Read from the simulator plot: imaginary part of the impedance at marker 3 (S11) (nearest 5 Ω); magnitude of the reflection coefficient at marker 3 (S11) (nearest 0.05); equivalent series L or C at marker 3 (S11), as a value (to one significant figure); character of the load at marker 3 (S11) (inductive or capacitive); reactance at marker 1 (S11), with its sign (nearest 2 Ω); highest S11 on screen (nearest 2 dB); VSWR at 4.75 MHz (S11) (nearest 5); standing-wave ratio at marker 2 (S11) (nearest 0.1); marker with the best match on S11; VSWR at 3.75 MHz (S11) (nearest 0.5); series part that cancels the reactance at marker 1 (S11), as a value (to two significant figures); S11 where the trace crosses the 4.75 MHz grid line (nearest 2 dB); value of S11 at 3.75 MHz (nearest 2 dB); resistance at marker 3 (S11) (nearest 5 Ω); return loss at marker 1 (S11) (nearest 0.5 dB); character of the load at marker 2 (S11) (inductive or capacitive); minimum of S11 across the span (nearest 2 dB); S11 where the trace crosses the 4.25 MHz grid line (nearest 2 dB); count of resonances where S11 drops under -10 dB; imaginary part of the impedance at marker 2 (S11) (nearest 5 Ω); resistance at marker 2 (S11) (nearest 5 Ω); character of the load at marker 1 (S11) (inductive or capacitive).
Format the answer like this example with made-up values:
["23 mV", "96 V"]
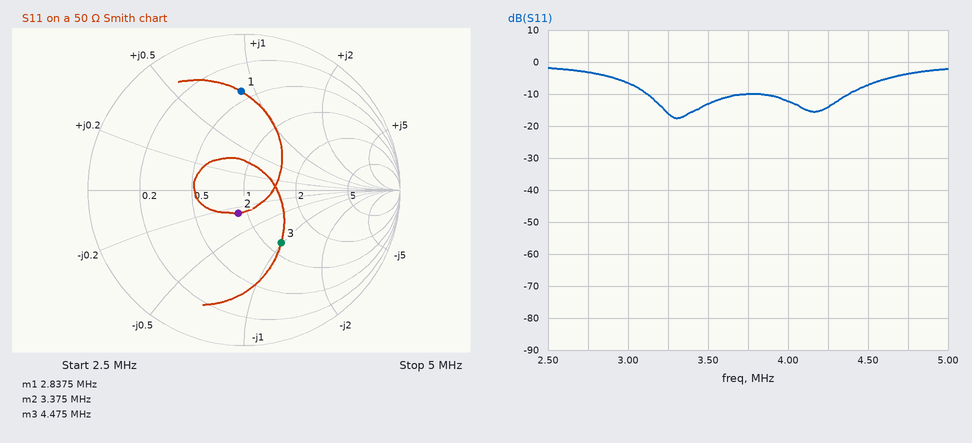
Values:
["-50 Ω", "0.40", "700 pF", "capacitive", "+44 Ω", "-2 dB", "5", "1.4", "marker 2", "2.0", "1.3 nF", "-4 dB", "-10 dB", "60 Ω", "4.0 dB", "capacitive", "-18 dB", "-14 dB", "2", "-15 Ω", "45 Ω", "inductive"]
